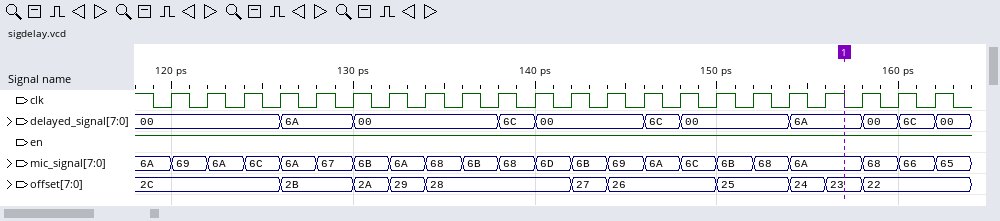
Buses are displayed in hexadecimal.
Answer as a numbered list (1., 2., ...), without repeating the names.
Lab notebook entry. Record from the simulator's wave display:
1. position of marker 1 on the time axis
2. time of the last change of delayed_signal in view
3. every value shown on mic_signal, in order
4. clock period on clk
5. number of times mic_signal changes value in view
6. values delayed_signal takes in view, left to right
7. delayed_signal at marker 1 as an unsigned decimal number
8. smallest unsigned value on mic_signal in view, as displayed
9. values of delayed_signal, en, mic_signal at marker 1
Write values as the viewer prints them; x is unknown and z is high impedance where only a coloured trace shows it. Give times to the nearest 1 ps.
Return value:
1. 157 ps
2. 162 ps
3. 6A, 69, 6A, 6C, 6A, 67, 6B, 6A, 68, 6B, 68, 6D, 6B, 69, 6A, 6C, 6B, 68, 6A, 68, 66, 65
4. 2 ps
5. 21
6. 00, 6A, 00, 6C, 00, 6C, 00, 6A, 00, 6C, 00
7. 106
8. 65
9. delayed_signal=6A, en=1, mic_signal=6A
